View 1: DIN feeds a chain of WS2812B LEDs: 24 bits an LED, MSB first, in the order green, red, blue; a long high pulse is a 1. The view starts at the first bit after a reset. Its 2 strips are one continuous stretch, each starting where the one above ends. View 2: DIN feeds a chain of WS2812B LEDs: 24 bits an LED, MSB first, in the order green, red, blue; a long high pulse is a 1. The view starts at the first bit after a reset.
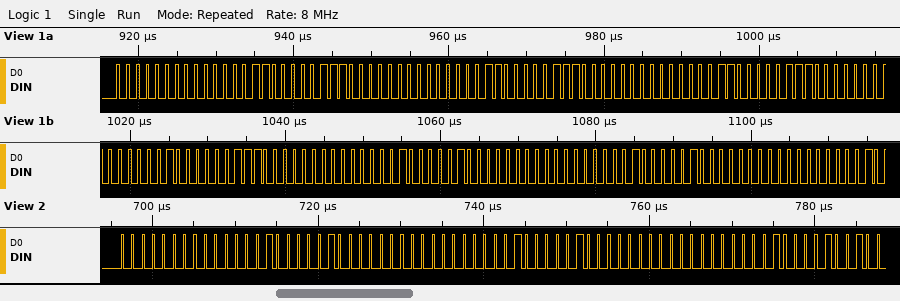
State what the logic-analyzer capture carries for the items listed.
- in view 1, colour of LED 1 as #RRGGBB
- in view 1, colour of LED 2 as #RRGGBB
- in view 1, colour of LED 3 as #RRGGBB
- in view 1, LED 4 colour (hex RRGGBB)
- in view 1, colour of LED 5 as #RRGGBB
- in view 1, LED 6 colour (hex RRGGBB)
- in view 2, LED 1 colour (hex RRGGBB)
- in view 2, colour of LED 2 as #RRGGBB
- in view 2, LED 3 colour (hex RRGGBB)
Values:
#030007
#030007
#030007
#020007
#020008
#020008
#020008
#020008
#010009
